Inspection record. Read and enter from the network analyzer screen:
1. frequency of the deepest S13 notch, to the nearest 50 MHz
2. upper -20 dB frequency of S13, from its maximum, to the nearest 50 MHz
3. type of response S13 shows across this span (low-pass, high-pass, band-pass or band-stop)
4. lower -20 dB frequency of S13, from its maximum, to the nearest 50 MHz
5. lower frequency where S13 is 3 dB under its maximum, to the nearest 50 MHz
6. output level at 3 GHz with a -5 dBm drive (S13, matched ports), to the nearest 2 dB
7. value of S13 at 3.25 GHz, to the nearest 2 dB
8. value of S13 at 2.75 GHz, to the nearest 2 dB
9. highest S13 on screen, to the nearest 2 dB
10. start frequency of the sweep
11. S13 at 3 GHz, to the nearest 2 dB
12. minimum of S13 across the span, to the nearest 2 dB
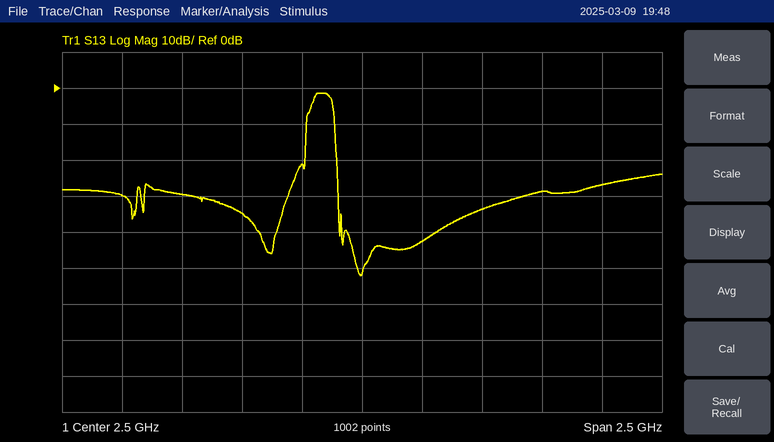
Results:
2.50 GHz
2.40 GHz
band-pass
2.25 GHz
2.30 GHz
-38 dBm
-28 dB
-42 dB
-2 dB
1.25 GHz
-34 dB
-52 dB
